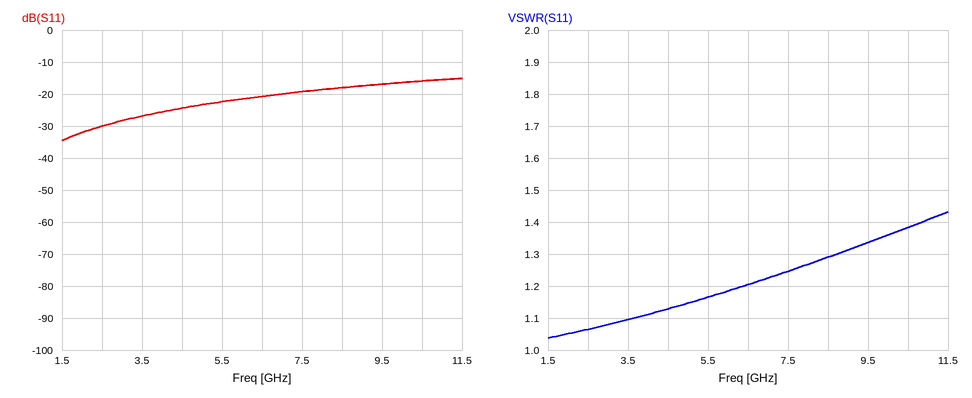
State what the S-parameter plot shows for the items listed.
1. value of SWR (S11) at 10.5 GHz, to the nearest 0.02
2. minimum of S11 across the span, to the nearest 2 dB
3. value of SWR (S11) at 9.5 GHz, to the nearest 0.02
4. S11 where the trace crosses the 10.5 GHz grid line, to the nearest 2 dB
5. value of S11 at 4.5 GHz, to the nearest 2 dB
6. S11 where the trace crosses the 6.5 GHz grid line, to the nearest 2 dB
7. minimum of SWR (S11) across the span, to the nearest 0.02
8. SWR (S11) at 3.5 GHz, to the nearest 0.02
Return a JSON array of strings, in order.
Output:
["1.38", "-34 dB", "1.34", "-16 dB", "-24 dB", "-20 dB", "1.04", "1.10"]
